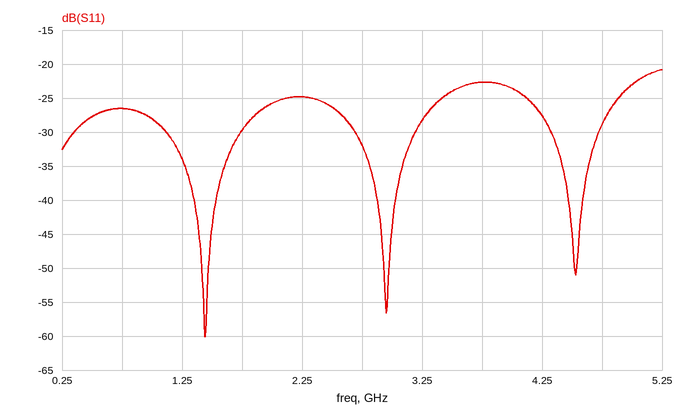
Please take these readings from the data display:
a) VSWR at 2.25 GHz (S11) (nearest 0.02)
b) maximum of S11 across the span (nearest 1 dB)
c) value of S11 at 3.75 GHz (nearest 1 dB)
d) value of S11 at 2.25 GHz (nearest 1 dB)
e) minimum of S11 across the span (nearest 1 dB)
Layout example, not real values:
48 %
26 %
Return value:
1.12
-21 dB
-23 dB
-25 dB
-60 dB
